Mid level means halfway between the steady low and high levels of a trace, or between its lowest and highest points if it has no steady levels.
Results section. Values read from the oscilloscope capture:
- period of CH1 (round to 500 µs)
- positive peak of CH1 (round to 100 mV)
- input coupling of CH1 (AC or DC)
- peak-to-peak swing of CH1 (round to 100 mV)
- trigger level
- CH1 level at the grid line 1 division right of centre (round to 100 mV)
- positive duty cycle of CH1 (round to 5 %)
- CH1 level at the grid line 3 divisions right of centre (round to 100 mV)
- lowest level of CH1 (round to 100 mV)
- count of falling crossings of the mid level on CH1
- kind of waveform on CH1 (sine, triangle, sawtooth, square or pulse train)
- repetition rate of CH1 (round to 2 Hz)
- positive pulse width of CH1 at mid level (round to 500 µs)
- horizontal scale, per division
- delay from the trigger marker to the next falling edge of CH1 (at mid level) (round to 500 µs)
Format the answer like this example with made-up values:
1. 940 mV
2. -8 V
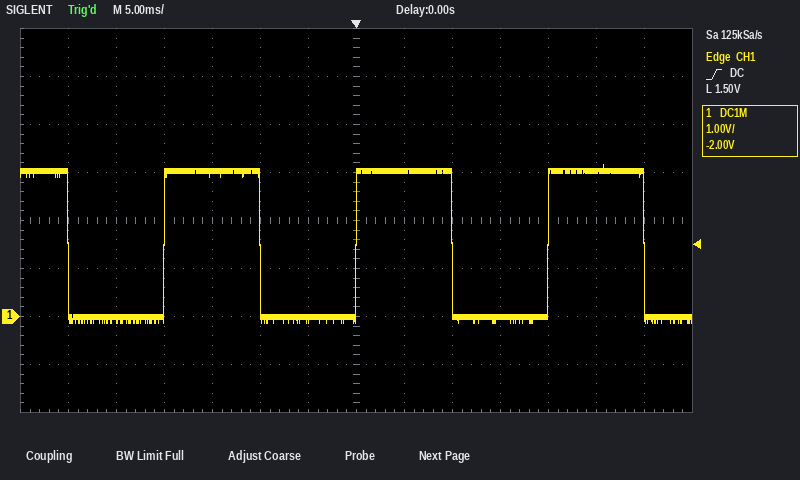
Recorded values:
1. 20.0 ms
2. 3.2 V
3. DC
4. 3.3 V
5. 1.50 V
6. 3.0 V
7. 50 %
8. 0.0 V
9. -100 mV
10. 4
11. square
12. 50 Hz
13. 10.0 ms
14. 5 ms
15. 10.0 ms
